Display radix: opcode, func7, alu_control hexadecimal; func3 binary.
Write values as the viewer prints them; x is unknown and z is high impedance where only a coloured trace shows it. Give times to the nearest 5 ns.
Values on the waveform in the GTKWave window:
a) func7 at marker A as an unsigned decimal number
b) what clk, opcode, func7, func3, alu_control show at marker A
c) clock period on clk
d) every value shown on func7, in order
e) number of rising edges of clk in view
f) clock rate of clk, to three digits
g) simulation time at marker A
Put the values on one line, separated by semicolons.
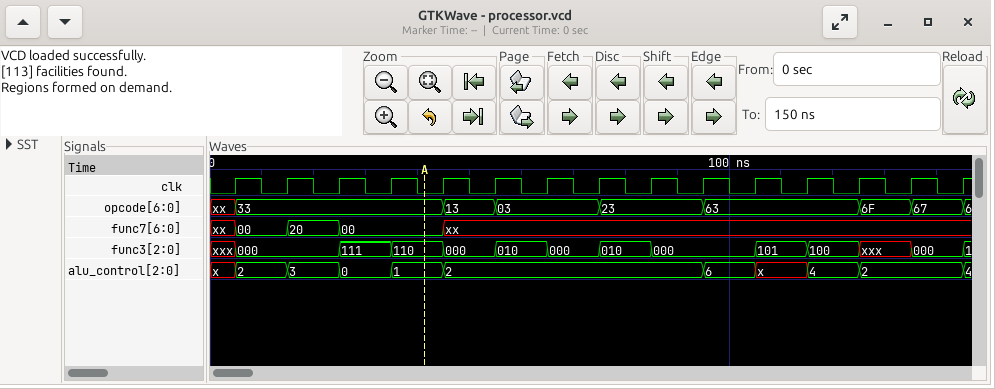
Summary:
0; clk=0, opcode=33, func7=00, func3=110, alu_control=1; 10 ns; xx, 00, 20, 00, xx; 15; 100 MHz; 40 ns
